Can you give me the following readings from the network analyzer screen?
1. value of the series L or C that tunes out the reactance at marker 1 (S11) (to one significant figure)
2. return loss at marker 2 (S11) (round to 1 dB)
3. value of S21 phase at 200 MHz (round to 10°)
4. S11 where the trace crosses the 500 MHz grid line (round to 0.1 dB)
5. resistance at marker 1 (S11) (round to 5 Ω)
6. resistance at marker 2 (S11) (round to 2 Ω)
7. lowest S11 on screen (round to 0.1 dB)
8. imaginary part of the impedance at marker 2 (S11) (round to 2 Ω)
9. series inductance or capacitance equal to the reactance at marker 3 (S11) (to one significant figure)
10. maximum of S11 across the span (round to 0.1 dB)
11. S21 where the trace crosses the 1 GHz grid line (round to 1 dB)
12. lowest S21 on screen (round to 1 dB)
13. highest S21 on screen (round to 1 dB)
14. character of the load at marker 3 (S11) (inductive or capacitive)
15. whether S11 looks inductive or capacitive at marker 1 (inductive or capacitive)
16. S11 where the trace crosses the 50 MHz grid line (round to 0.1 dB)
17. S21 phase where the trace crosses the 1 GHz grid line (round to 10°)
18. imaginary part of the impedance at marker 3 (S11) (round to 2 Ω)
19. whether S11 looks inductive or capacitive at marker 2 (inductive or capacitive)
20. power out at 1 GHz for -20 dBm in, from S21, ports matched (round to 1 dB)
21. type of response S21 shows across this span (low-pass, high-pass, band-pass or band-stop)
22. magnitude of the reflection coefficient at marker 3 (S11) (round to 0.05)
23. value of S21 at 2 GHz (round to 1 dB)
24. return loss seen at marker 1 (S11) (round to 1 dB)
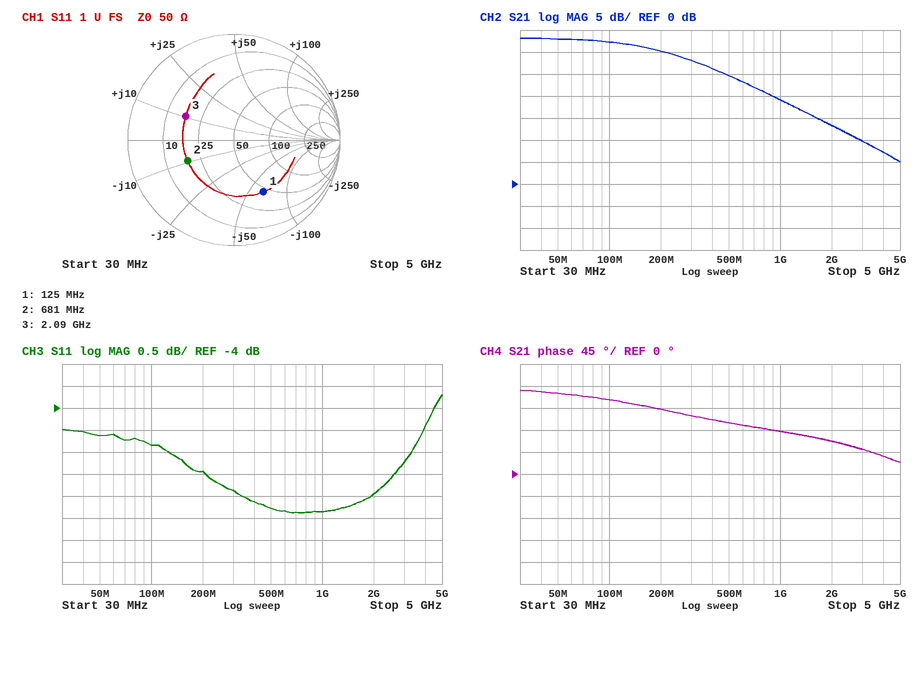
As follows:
80 nH
6 dB
130°
-6.3 dB
45 Ω
18 Ω
-6.4 dB
-10 Ω
800 pH
-3.7 dB
19 dB
5 dB
33 dB
inductive
capacitive
-4.6 dB
90°
+10 Ω
capacitive
-1 dBm
low-pass
0.50
13 dB
5 dB
